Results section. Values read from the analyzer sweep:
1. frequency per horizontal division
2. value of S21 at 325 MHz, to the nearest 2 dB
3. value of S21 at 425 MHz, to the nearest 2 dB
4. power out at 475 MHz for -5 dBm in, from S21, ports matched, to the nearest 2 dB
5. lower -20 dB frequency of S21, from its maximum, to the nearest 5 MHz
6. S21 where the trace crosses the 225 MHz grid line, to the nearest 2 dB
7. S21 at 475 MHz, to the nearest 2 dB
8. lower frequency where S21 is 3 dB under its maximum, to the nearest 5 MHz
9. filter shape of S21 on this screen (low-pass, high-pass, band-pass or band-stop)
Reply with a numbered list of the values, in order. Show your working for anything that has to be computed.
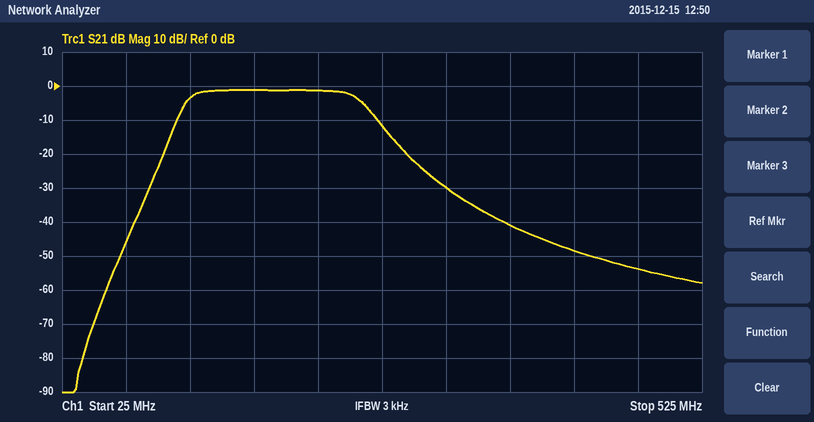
1. 50 MHz
2. -30 dB
3. -48 dB
4. -5 dBm + (-54 dB) = -58 dBm
5. 105 MHz
6. -2 dB
7. -54 dB
8. 125 MHz
9. band-pass
